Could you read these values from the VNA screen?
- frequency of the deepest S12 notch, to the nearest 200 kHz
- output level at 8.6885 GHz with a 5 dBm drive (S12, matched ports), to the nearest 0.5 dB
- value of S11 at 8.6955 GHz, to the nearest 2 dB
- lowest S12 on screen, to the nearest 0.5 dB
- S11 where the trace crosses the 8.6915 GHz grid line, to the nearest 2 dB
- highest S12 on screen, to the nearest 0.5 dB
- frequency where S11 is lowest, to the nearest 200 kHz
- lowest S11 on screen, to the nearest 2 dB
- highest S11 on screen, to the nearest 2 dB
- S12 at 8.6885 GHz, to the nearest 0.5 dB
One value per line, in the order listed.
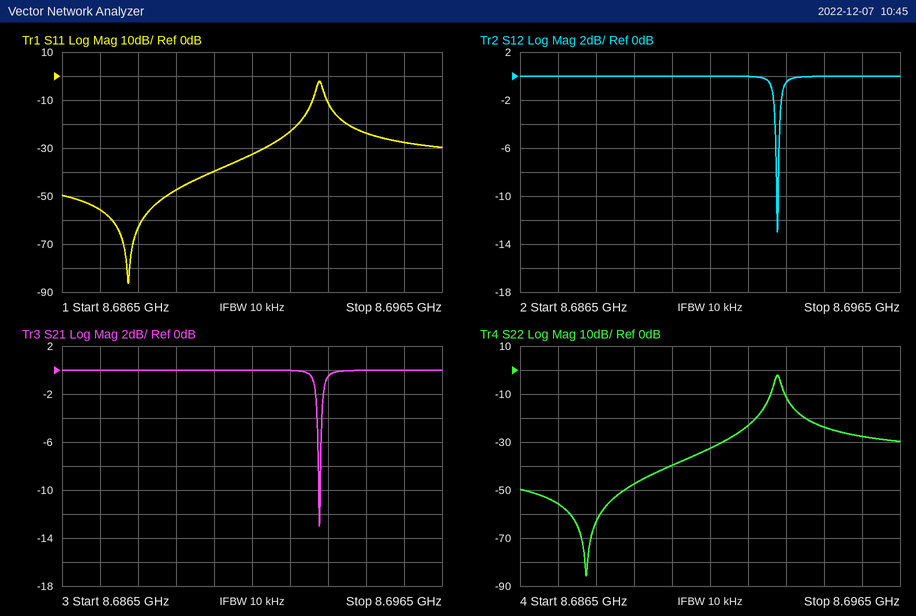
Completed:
8.6932 GHz
5.0 dBm
-28 dB
-13.0 dB
-32 dB
0.0 dB
8.6882 GHz
-86 dB
-2 dB
0.0 dB
